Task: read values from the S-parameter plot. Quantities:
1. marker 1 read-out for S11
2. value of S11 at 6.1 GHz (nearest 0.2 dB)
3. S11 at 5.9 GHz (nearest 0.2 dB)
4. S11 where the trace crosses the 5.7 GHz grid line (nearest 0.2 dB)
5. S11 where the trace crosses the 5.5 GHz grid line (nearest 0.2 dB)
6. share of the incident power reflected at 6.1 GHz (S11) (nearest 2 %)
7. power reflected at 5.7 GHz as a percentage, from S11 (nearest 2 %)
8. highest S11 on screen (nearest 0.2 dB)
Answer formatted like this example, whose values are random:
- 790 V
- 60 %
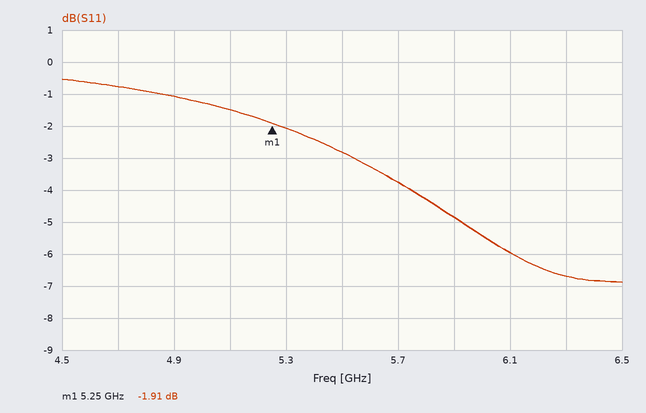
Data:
- -1.91 dB
- -6.0 dB
- -4.8 dB
- -3.8 dB
- -2.8 dB
- 26 %
- 42 %
- -0.6 dB
